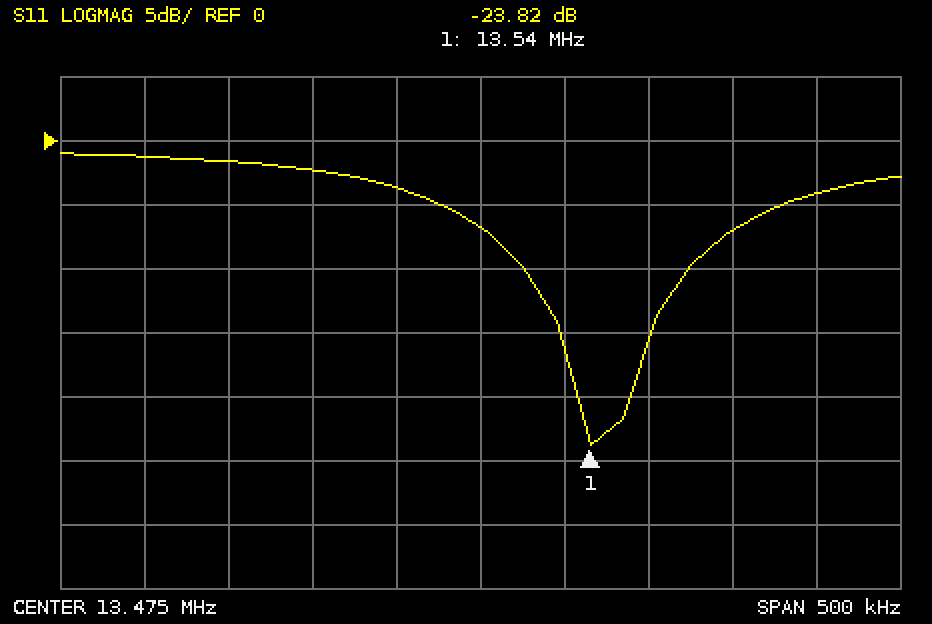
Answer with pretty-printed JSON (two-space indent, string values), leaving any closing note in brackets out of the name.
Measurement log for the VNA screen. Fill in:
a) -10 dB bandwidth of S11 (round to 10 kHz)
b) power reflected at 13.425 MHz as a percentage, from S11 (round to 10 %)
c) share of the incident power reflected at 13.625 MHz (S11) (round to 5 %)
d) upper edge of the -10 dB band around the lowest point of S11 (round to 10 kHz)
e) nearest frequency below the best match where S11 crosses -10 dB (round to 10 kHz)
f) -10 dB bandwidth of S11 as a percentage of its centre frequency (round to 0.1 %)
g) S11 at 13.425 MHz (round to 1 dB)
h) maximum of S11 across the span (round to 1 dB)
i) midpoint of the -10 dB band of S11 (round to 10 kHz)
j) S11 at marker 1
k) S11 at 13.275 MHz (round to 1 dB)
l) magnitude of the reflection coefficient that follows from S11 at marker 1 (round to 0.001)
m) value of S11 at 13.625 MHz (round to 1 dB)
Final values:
{
  "-10 dB bandwidth of S11": "100 kHz",
  "power reflected at 13.425 MHz as a percentage, from S11": "40 %",
  "share of the incident power reflected at 13.625 MHz (S11)": "20 %",
  "upper edge of the -10 dB band around the lowest point of S11": "13.60 MHz",
  "nearest frequency below the best match where S11 crosses -10 dB": "13.50 MHz",
  "-10 dB bandwidth of S11 as a percentage of its centre frequency": "0.7 %",
  "S11 at 13.425 MHz": "-4 dB",
  "maximum of S11 across the span": "-1 dB",
  "midpoint of the -10 dB band of S11": "13.55 MHz",
  "S11 at marker 1": "-23.82 dB",
  "S11 at 13.275 MHz": "-1 dB",
  "magnitude of the reflection coefficient that follows from S11 at marker 1": "0.064",
  "value of S11 at 13.625 MHz": "-7 dB"
}
